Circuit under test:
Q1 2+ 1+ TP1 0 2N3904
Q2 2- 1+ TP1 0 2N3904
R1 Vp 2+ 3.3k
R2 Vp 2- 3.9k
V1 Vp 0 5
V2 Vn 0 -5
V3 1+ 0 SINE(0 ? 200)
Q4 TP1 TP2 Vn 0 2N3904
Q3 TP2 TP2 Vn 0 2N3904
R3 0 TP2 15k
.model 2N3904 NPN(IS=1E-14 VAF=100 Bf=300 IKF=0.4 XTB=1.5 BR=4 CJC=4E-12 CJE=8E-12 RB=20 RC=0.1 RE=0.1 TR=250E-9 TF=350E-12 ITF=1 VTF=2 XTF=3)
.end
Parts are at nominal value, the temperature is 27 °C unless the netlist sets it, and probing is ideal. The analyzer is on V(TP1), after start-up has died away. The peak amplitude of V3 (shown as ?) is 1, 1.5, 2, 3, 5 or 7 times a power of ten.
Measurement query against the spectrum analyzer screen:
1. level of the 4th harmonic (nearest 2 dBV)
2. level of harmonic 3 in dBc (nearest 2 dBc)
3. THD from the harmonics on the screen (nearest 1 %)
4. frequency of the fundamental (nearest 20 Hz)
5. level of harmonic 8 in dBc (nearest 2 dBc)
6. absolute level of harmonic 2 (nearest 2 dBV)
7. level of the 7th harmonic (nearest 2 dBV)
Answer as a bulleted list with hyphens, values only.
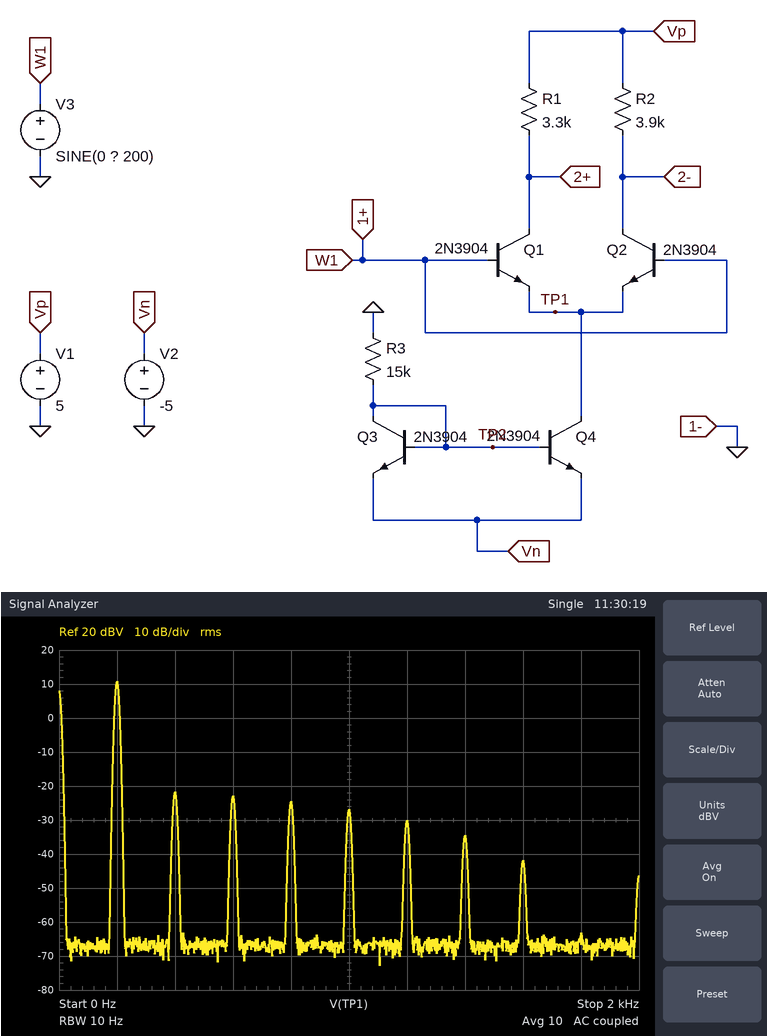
- -24 dBV
- -34 dBc
- 4 %
- 200 Hz
- -52 dBc
- -22 dBV
- -34 dBV
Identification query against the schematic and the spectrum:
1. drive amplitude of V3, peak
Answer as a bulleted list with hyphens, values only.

- 5 V
